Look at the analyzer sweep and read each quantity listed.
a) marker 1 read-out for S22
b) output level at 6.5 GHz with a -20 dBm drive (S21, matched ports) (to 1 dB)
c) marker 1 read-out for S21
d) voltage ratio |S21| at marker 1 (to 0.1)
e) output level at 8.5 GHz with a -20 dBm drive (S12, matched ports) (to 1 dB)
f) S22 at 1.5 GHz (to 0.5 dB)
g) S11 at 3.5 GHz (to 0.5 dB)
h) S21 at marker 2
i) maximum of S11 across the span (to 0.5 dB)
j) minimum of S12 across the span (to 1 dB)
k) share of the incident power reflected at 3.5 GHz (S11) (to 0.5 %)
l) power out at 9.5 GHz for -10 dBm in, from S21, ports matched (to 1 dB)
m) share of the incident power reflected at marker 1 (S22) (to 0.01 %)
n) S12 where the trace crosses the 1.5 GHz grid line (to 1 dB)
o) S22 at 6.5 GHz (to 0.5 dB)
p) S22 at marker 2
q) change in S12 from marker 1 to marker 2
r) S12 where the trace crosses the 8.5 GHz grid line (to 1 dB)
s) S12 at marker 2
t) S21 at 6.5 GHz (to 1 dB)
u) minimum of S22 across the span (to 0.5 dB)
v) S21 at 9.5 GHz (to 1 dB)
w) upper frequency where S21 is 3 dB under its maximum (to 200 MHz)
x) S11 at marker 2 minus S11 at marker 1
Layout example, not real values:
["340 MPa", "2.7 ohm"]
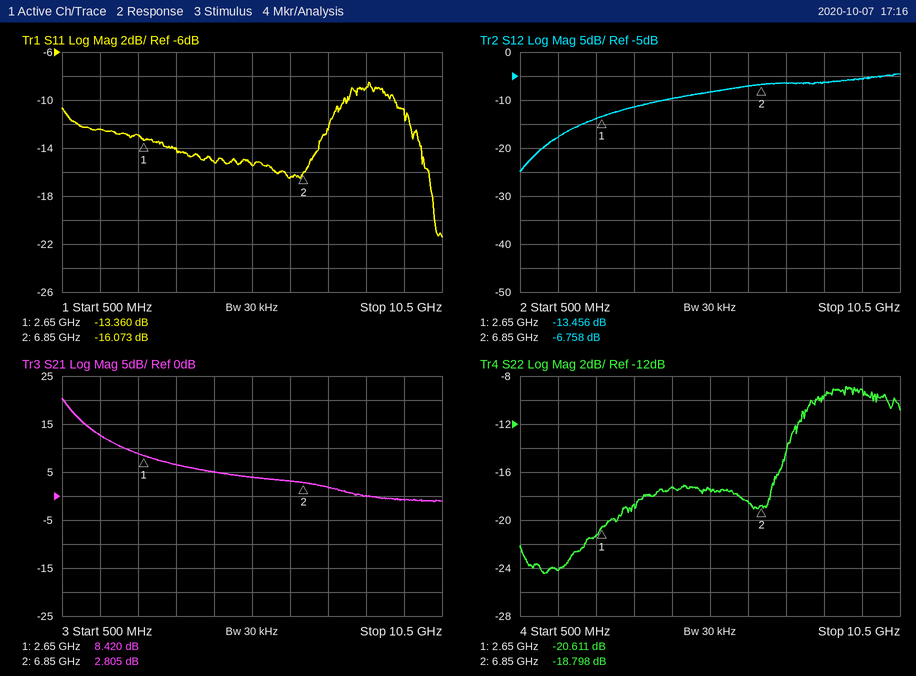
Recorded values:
["-20.611 dB", "-17 dBm", "8.420 dB", "2.6", "-26 dBm", "-24.0 dB", "-14.0 dB", "2.805 dB", "-8.5 dB", "-25 dB", "4.0 %", "-11 dBm", "0.87 %", "-18 dB", "-18.5 dB", "-18.798 dB", "6.698 dB", "-6 dB", "-6.758 dB", "3 dB", "-24.5 dB", "-1 dB", "800 MHz", "-2.713 dB"]
